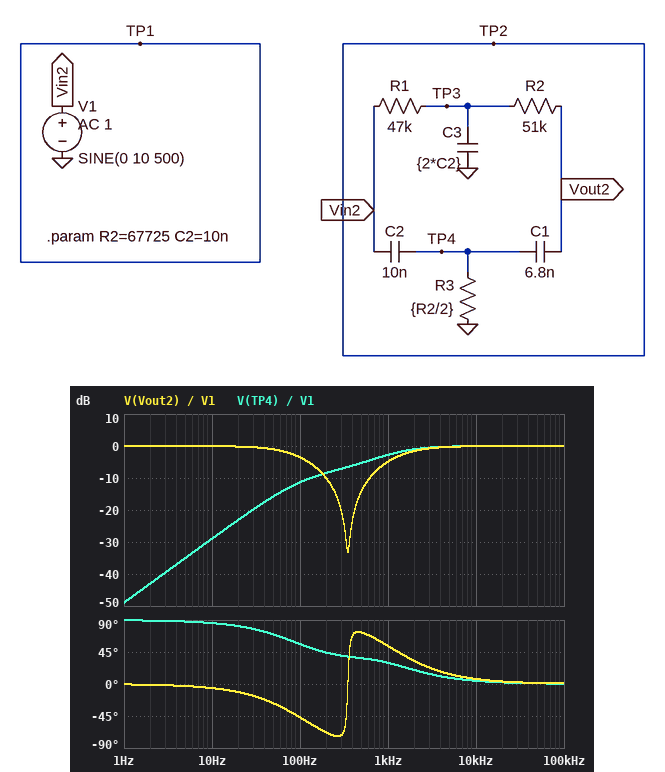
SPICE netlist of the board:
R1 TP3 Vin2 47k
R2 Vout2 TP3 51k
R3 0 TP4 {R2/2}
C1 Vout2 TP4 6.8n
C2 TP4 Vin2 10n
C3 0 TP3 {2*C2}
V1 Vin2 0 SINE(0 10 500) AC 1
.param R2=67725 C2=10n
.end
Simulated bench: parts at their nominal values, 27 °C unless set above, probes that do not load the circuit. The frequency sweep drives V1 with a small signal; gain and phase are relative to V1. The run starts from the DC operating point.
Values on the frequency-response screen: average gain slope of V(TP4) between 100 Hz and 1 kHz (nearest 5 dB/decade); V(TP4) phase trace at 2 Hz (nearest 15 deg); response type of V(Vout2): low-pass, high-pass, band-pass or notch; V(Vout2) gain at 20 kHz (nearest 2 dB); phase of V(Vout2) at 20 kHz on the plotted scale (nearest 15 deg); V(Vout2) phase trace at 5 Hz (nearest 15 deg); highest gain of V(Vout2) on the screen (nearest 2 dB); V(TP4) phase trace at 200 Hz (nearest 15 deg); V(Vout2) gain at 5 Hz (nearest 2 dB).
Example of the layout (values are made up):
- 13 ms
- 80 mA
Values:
- 10 dB/decade
- 90 deg
- notch
- 0 dB
- 0 deg
- 0 deg
- 0 dB
- 45 deg
- 0 dB
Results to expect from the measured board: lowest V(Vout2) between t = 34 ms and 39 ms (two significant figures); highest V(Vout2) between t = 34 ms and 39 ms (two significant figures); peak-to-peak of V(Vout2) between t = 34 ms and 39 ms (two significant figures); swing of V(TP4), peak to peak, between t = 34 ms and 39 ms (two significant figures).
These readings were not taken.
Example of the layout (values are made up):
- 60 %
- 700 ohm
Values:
- -2.0 V
- 2.0 V
- 4.0 V
- 11 V
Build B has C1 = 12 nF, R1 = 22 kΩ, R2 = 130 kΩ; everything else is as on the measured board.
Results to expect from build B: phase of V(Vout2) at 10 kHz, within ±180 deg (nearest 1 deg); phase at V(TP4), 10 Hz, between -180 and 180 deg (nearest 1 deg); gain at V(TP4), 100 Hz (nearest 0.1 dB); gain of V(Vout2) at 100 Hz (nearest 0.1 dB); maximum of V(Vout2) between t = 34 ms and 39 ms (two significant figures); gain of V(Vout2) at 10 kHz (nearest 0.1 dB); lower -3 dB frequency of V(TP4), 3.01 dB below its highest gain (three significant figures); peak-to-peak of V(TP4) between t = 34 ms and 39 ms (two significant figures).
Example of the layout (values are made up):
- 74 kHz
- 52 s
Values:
- 4 deg
- 83 deg
- -11.3 dB
- -6.7 dB
- 4.6 V
- 0 dB
- 695 Hz
- 12 V
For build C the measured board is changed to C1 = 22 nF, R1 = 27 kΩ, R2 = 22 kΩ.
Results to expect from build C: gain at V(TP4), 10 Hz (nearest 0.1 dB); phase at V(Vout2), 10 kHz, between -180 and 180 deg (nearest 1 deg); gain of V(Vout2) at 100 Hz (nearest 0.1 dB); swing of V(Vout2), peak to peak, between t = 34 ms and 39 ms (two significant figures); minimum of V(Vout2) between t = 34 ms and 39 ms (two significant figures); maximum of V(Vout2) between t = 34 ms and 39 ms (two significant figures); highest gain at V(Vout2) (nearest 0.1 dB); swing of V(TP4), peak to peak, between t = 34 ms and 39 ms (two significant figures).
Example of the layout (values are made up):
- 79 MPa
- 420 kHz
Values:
- -23.4 dB
- 9 deg
- -4.2 dB
- 4.3 V
- -2.2 V
- 2.2 V
- 0 dB
- 8.8 V
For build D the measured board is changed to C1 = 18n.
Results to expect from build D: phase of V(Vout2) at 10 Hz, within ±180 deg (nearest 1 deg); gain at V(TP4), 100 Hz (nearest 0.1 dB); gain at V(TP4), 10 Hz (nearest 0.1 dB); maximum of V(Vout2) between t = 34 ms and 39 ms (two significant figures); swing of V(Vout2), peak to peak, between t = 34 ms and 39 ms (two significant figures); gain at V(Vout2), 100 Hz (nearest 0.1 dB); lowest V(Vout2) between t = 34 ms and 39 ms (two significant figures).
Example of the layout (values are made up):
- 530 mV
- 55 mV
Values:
- -10 deg
- -10.9 dB
- -24.6 dB
- 3.5 V
- 7.0 V
- -7.6 dB
- -3.5 V
